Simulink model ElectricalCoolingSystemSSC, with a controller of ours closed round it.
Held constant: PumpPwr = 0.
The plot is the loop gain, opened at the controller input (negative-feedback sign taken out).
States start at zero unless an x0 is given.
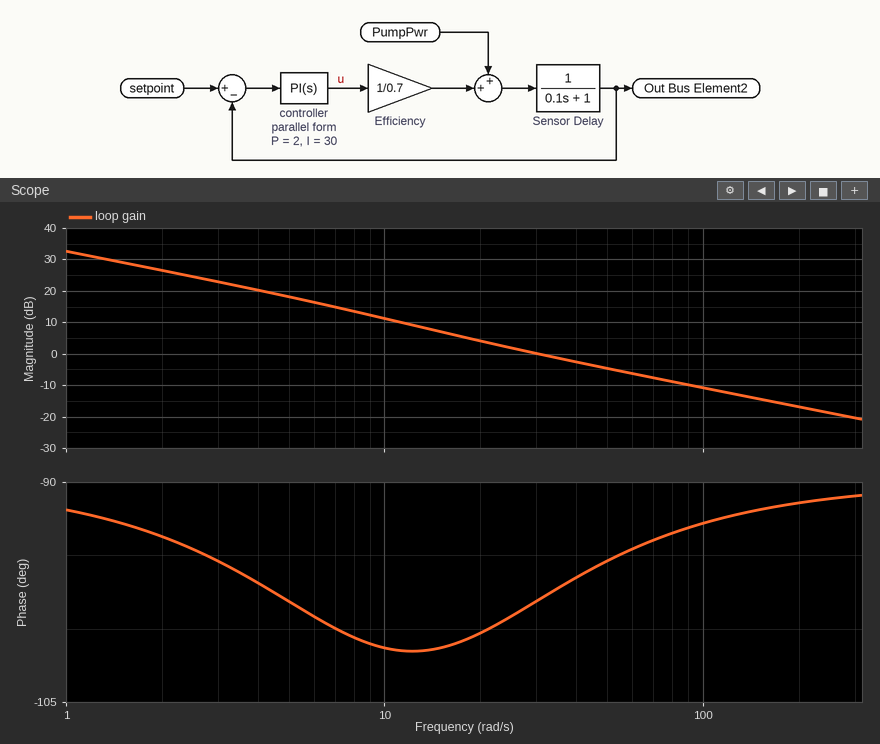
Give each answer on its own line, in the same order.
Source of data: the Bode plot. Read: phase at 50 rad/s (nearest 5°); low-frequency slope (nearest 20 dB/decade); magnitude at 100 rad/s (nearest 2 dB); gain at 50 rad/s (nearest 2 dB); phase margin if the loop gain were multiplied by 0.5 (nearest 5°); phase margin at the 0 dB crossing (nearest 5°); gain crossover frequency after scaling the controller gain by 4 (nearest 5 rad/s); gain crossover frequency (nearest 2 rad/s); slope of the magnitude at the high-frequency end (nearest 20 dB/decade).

-95°
-20 dB/decade
-10 dB
-4 dB
80°
80°
115 rad/s
30 rad/s
-20 dB/decade
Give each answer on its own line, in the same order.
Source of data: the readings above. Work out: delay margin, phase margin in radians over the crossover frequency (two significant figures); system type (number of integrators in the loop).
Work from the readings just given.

0.047 s
1
